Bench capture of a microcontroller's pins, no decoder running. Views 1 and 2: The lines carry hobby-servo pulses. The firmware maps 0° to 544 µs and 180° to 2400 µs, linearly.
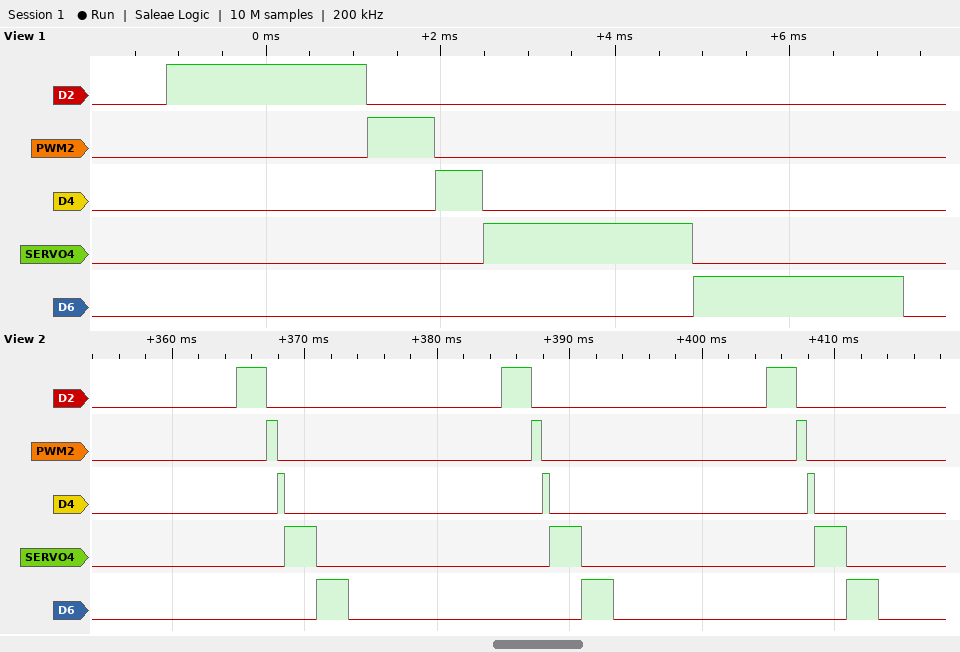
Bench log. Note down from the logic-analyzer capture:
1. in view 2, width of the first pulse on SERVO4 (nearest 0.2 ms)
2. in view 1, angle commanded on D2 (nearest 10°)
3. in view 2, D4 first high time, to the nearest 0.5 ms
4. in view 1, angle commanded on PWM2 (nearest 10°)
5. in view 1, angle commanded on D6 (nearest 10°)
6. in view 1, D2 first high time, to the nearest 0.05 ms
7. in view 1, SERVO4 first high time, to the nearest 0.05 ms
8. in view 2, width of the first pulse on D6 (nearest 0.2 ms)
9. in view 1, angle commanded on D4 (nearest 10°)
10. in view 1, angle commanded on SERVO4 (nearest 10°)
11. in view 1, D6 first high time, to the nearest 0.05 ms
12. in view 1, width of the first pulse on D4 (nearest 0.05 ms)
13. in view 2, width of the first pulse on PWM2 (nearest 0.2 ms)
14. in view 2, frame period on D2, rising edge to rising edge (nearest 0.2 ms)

2.4 ms
170°
0.5 ms
20°
180°
2.30 ms
2.40 ms
2.4 ms
0°
180°
2.40 ms
0.55 ms
0.8 ms
20.0 ms
